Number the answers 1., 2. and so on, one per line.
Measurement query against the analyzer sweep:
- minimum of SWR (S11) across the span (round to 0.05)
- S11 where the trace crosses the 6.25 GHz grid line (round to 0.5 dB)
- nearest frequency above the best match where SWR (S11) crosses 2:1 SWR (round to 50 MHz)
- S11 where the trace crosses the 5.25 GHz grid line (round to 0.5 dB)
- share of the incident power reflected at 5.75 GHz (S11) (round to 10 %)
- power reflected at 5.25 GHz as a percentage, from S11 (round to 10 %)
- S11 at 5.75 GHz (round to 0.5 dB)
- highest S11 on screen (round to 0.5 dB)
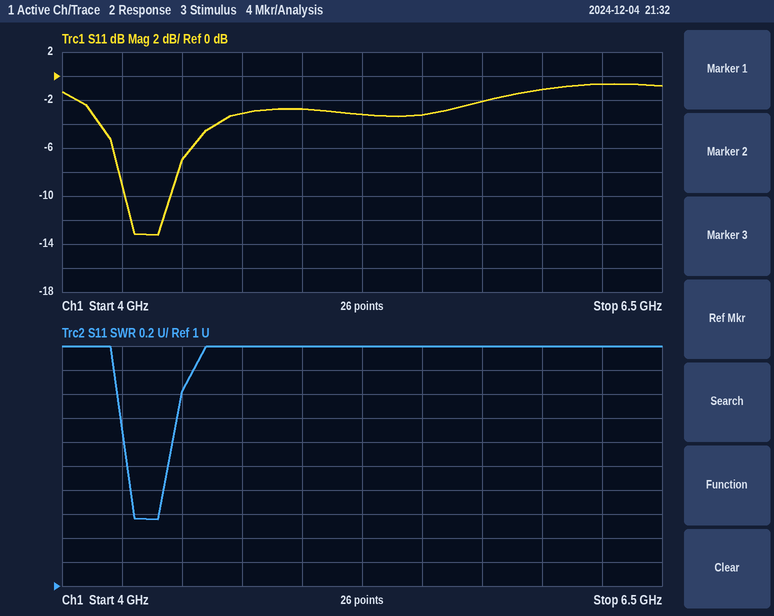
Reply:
1. 1.55
2. -0.5 dB
3. 4.45 GHz
4. -3.0 dB
5. 60 %
6. 50 %
7. -2.0 dB
8. -0.5 dB
